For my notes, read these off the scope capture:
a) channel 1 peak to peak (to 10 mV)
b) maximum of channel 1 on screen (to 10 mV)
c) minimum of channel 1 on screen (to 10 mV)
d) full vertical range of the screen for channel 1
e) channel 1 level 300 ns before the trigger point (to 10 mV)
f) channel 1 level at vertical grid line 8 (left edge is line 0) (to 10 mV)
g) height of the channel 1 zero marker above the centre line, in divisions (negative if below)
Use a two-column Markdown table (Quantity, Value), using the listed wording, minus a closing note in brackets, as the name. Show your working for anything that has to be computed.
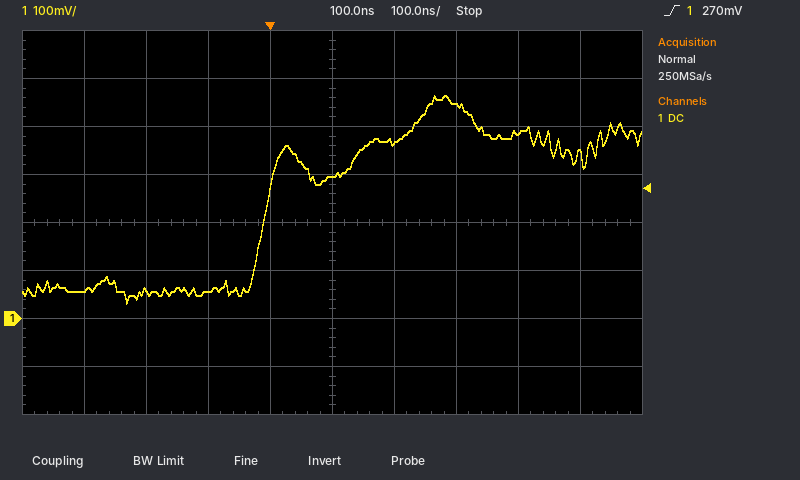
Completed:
| Quantity | Value |
|---|---|
| channel 1 peak to peak | 460 mV − (30 mV) = 430 mV |
| maximum of channel 1 on screen | 460 mV |
| minimum of channel 1 on screen | 30 mV |
| full vertical range of the screen for channel 1 | 800 mV |
| channel 1 level 300 ns before the trigger point | 60 mV |
| channel 1 level at vertical grid line 8 (left edge is line 0) | 390 mV |
| height of the channel 1 zero marker above the centre line, in divisions | -2.0 div |
